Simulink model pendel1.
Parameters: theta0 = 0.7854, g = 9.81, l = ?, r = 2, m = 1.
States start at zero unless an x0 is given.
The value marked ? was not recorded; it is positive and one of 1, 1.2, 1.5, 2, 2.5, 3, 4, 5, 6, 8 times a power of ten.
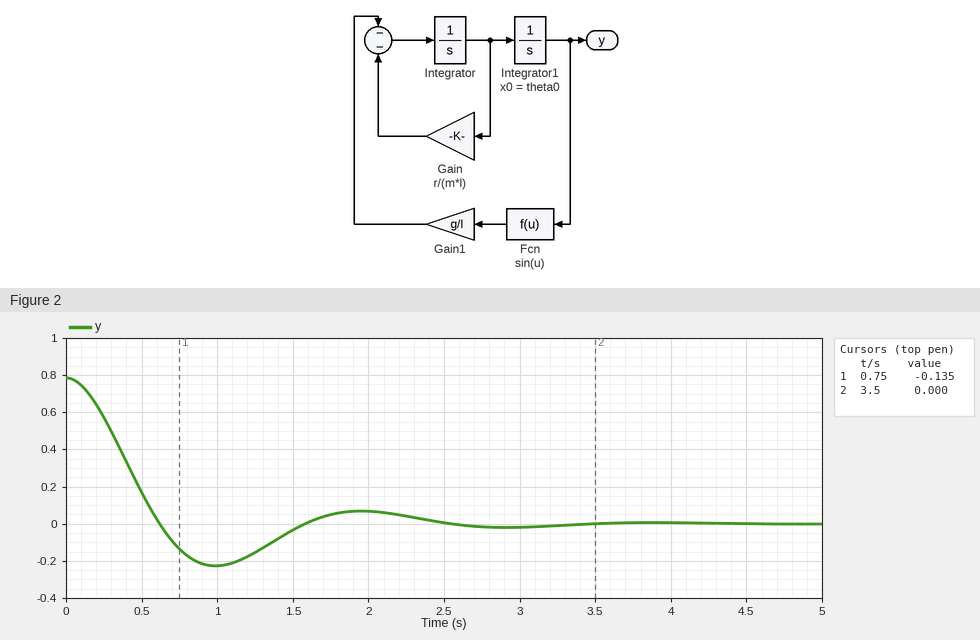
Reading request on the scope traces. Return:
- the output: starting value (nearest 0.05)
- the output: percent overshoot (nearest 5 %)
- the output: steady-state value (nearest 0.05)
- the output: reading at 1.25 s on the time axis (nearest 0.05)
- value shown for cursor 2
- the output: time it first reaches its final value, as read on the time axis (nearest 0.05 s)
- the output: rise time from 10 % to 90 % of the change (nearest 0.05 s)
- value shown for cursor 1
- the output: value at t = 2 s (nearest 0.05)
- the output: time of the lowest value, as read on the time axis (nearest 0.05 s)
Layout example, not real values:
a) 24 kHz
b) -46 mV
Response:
a) 0.80
b) 30 %
c) 0.00
d) -0.15
e) 0.000
f) 0.60 s
g) 0.40 s
h) -0.135
i) 0.05
j) 1.00 s
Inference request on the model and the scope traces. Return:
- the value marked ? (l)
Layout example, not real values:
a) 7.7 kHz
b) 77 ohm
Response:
a) 0.8
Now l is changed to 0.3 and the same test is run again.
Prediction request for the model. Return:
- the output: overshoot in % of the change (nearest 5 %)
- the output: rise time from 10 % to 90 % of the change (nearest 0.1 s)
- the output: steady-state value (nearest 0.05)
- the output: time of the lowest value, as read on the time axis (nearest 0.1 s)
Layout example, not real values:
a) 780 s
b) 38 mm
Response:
a) 10 %
b) 0.3 s
c) 0.00
d) 0.7 s
